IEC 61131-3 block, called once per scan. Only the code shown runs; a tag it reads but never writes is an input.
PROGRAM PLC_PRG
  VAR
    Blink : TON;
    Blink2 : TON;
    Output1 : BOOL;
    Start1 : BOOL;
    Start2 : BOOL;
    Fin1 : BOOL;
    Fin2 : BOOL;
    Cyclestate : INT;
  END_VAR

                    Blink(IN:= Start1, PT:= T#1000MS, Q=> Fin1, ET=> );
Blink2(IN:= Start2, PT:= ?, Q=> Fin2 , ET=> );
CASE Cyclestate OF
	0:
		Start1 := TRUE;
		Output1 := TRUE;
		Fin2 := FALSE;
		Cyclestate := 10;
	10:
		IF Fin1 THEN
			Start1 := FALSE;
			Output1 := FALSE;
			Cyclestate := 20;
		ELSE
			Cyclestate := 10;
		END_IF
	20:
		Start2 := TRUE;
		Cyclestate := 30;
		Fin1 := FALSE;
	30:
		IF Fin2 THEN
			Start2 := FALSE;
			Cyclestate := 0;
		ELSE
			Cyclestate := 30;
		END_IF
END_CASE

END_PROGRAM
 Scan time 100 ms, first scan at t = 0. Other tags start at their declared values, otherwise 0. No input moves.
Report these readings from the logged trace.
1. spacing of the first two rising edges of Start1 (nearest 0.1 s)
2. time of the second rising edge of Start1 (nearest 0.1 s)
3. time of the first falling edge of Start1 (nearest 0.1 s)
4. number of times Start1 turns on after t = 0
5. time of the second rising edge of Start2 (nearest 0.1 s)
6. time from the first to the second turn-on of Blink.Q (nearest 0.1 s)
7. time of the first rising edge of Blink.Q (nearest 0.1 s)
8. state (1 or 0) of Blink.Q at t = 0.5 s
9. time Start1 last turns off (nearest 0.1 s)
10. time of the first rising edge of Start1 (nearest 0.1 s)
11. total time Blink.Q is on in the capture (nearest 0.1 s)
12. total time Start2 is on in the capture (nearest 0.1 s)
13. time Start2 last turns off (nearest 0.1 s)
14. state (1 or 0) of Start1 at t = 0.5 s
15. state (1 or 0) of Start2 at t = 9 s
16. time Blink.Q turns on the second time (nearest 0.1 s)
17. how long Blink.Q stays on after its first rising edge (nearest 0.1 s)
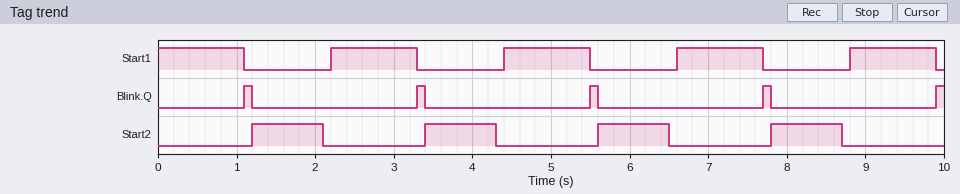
2.2 s
4.4 s
1.1 s
4
3.4 s
2.2 s
1.1 s
0
9.9 s
2.2 s
0.5 s
3.6 s
8.7 s
1
0
3.3 s
0.1 s
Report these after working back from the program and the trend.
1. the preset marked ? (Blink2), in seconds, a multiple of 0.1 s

0.8 s
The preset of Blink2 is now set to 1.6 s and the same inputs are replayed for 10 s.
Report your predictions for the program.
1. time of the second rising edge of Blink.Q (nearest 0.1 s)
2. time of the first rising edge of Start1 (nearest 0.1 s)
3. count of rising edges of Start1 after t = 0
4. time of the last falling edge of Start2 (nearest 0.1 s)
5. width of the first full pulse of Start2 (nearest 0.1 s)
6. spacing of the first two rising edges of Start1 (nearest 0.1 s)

4.1 s
3.0 s
3
8.9 s
1.7 s
3.0 s
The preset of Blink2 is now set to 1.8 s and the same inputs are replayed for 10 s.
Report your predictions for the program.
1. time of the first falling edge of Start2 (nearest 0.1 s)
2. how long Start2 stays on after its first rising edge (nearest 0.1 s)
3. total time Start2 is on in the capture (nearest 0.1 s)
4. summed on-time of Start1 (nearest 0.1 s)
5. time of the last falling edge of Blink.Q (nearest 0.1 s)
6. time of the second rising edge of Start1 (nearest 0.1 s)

3.1 s
1.9 s
5.7 s
3.7 s
7.6 s
6.4 s
